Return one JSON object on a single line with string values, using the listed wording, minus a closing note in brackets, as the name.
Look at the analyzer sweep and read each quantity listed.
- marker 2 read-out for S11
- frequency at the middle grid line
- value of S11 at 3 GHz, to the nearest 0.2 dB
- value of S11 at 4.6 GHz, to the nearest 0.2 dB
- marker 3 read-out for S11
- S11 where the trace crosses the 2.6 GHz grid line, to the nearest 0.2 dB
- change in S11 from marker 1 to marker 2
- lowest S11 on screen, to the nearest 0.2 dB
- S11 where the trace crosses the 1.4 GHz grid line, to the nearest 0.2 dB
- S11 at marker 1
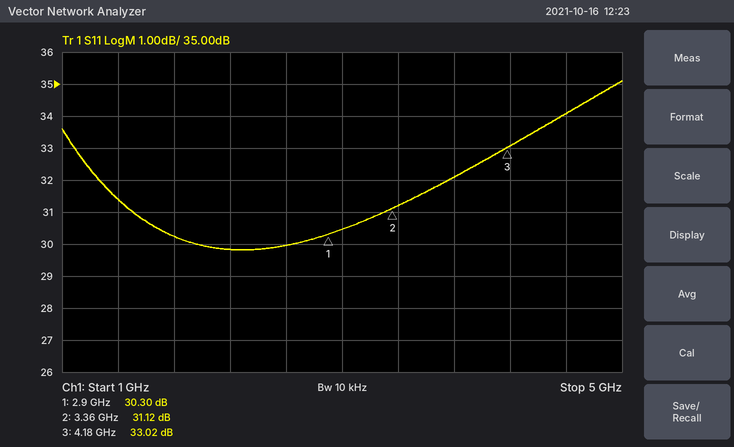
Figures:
{"marker 2 read-out for S11": "31.12 dB", "frequency at the middle grid line": "3 GHz", "value of S11 at 3 GHz, to the nearest 0.2 dB": "30.4 dB", "value of S11 at 4.6 GHz, to the nearest 0.2 dB": "34.0 dB", "marker 3 read-out for S11": "33.02 dB", "S11 where the trace crosses the 2.6 GHz grid line, to the nearest 0.2 dB": "30.0 dB", "change in S11 from marker 1 to marker 2": "0.82 dB", "lowest S11 on screen, to the nearest 0.2 dB": "29.8 dB", "S11 where the trace crosses the 1.4 GHz grid line, to the nearest 0.2 dB": "31.4 dB", "S11 at marker 1": "30.30 dB"}
